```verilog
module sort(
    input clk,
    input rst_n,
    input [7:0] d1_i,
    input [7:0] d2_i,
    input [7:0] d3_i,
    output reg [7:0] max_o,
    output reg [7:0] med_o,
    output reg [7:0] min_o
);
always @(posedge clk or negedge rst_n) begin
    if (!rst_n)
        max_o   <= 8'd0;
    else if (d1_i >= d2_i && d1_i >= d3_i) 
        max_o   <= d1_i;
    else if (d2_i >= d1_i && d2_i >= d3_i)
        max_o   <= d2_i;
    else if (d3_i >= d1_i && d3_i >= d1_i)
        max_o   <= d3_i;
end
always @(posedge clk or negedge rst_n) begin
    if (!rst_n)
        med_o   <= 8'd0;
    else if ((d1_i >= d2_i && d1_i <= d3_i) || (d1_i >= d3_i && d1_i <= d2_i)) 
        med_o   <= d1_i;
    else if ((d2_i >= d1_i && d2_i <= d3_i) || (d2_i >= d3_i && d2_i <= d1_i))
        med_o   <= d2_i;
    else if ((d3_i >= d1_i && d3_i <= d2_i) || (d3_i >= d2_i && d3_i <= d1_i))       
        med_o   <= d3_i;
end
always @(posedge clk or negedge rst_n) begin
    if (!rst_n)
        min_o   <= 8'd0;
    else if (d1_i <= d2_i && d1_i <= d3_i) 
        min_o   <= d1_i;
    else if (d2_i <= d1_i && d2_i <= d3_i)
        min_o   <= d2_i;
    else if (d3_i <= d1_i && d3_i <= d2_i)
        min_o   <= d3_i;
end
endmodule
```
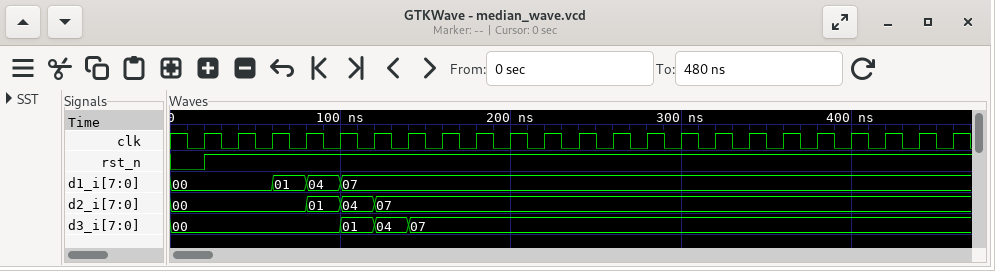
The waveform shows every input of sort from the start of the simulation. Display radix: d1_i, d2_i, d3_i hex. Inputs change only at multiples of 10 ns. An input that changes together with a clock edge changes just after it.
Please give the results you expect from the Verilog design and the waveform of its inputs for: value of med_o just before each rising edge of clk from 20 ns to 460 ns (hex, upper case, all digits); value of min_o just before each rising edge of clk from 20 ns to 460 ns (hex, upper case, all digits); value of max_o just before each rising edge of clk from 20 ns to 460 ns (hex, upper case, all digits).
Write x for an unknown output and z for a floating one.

00, 00, 00, 00, 00, 01, 04, 07, 07, 07, 07, 07, 07, 07, 07, 07, 07, 07, 07, 07, 07, 07, 07
00, 00, 00, 00, 00, 00, 01, 04, 07, 07, 07, 07, 07, 07, 07, 07, 07, 07, 07, 07, 07, 07, 07
00, 00, 00, 00, 01, 04, 07, 07, 07, 07, 07, 07, 07, 07, 07, 07, 07, 07, 07, 07, 07, 07, 07
